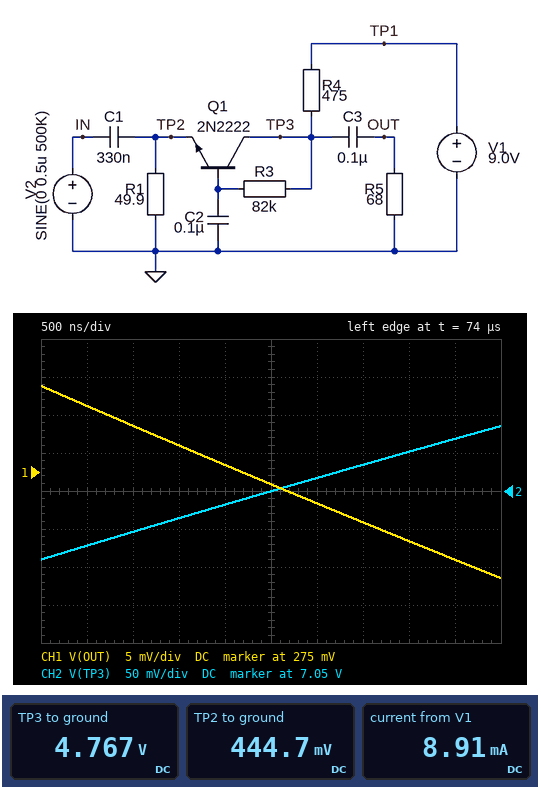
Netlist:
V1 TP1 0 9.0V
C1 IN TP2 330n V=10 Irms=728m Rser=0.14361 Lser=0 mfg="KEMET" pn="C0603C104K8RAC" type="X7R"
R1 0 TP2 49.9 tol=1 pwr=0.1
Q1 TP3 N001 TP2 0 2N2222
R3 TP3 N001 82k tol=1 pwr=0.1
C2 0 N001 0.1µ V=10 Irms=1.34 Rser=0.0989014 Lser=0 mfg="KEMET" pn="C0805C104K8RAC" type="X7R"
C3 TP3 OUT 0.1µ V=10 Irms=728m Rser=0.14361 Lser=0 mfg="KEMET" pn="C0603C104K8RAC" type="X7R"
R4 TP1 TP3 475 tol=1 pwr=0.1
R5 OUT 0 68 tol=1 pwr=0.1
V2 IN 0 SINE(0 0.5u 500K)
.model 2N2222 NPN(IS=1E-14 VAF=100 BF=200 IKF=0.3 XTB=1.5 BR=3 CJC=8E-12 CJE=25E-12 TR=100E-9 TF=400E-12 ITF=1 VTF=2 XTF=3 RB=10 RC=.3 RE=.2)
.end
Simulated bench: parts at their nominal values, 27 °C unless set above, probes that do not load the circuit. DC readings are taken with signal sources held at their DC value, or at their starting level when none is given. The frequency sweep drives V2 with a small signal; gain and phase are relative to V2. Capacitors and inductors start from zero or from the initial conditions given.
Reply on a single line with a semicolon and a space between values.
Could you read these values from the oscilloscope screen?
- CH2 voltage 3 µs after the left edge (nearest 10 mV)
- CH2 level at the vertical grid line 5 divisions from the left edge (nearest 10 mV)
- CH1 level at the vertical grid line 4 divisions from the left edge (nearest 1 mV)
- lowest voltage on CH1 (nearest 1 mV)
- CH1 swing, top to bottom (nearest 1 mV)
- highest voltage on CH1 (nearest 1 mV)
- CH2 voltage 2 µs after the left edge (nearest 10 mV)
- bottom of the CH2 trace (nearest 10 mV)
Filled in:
7.07 V; 7.05 V; 276 mV; 261 mV; 25 mV; 286 mV; 7.03 V; 6.96 V
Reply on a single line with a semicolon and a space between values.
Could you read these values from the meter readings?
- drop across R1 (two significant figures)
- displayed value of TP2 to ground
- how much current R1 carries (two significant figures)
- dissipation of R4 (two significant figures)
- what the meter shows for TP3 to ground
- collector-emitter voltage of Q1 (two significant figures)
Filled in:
440 mV; 444.7 mV; 8.9 mA; 38 mW; 4.767 V; 4.3 V
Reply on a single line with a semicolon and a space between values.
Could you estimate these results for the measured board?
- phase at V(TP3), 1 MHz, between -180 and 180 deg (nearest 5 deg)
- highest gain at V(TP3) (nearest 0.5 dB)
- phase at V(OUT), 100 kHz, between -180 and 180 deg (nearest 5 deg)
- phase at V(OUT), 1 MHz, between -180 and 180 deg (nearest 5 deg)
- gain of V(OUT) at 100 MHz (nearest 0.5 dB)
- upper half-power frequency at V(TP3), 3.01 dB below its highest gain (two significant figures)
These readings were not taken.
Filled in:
5 deg; 25.0 dB; 60 deg; 10 deg; 19.0 dB; 62 MHz
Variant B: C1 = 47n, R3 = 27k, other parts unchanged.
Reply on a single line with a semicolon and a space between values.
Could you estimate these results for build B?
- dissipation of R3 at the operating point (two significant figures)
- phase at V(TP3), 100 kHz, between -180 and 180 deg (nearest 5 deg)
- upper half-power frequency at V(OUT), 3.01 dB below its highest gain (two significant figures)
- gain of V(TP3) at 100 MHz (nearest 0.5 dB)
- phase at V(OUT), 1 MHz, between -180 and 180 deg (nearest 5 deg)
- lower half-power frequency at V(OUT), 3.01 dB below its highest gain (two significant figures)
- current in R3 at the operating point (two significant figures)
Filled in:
110 µW; 75 deg; 48 MHz; 19.5 dB; 55 deg; 1.3 MHz; 64 µA
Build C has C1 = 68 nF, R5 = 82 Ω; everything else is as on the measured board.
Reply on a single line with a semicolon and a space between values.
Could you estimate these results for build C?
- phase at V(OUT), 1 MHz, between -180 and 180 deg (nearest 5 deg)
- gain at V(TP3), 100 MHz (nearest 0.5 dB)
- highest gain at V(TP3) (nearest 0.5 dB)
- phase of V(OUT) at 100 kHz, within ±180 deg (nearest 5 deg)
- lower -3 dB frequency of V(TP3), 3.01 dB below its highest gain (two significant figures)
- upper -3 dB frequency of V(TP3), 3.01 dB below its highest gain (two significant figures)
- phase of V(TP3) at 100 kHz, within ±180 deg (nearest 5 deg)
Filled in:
35 deg; 20.0 dB; 26.0 dB; 85 deg; 720 kHz; 59 MHz; 75 deg
